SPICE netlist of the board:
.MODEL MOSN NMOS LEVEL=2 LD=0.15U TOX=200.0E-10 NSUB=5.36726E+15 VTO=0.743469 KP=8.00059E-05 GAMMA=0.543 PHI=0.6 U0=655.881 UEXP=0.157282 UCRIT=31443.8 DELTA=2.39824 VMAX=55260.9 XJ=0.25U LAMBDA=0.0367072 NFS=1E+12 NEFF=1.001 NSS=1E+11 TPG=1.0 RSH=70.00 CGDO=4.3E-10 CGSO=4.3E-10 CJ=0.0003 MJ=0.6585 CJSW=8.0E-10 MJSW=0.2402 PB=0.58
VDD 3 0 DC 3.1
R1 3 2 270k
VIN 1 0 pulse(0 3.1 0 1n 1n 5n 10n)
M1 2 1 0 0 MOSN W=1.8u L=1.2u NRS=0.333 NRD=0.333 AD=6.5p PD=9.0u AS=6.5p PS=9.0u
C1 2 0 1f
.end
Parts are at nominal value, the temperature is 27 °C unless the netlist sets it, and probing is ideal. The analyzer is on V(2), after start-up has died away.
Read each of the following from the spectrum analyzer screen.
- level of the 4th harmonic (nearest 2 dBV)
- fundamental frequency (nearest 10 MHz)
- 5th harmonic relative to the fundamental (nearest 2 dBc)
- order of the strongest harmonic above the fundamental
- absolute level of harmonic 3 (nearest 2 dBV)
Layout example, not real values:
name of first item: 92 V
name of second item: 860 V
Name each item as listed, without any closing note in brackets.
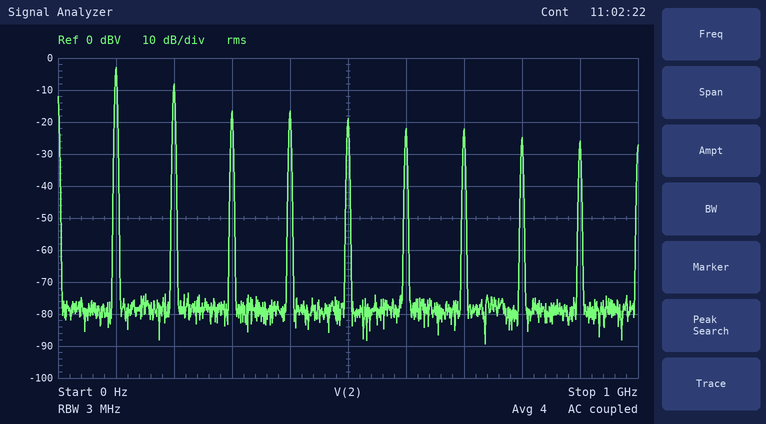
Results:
level of the 4th harmonic: -16 dBV
fundamental frequency: 100 MHz
5th harmonic relative to the fundamental: -16 dBc
order of the strongest harmonic above the fundamental: 2
absolute level of harmonic 3: -16 dBV
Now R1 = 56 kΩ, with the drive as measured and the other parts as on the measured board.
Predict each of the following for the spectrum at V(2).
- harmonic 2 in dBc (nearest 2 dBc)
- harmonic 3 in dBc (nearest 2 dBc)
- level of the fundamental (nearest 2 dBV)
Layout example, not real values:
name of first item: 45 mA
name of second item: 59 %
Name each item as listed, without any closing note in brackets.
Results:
harmonic 2 in dBc: -8 dBc
harmonic 3 in dBc: -18 dBc
level of the fundamental: 2 dBV
